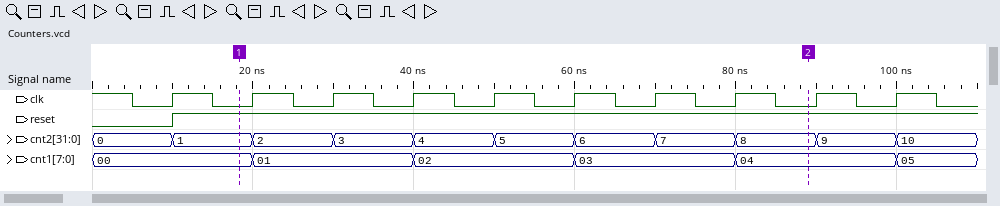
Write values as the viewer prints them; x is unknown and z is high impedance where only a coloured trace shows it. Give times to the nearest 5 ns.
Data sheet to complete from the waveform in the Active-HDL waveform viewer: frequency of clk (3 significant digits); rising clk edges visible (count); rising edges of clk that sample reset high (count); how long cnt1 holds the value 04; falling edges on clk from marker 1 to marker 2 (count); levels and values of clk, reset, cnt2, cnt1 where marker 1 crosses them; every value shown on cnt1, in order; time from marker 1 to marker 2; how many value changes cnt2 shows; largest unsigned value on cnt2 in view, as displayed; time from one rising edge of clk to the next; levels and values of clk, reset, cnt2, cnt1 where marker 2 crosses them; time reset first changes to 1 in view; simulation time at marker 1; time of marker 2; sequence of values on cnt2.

100 MHz
10
9
20 ns
7
clk=0, reset=1, cnt2=1, cnt1=00
00, 01, 02, 03, 04, 05
70 ns
10
10
10 ns
clk=0, reset=1, cnt2=8, cnt1=04
10 ns
20 ns
90 ns
0, 1, 2, 3, 4, 5, 6, 7, 8, 9, 10
